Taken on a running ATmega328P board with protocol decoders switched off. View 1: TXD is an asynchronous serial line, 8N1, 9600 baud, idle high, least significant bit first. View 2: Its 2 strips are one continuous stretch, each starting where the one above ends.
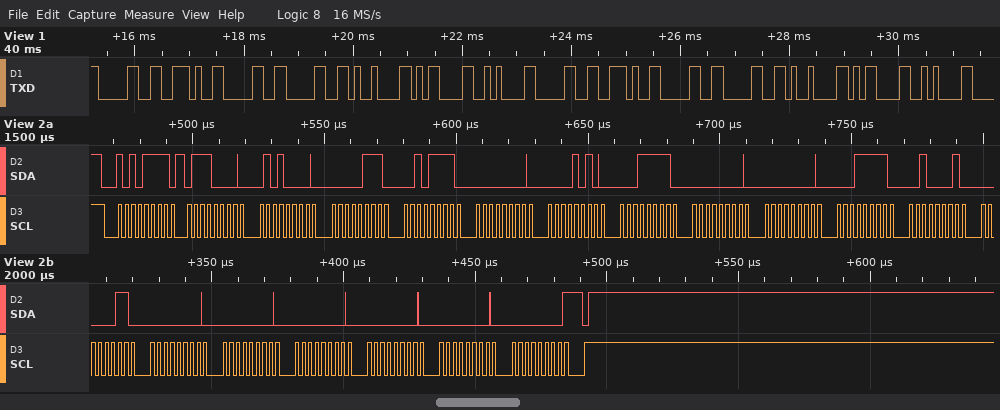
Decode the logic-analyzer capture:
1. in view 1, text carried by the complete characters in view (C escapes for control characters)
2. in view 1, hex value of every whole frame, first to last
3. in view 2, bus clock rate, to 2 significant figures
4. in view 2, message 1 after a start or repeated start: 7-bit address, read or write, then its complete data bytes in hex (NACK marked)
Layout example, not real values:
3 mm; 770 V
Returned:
"0.00\t\r\n0.00\t\r\n"; 30 2E 30 30 09 0D 0A 30 2E 30 30 09 0D 0A; 400 kHz; 0x57 read: 70 50 07 2F 00 0A 1F 00 00 1F 21 03 00 00 00 00 00 00 NACK
